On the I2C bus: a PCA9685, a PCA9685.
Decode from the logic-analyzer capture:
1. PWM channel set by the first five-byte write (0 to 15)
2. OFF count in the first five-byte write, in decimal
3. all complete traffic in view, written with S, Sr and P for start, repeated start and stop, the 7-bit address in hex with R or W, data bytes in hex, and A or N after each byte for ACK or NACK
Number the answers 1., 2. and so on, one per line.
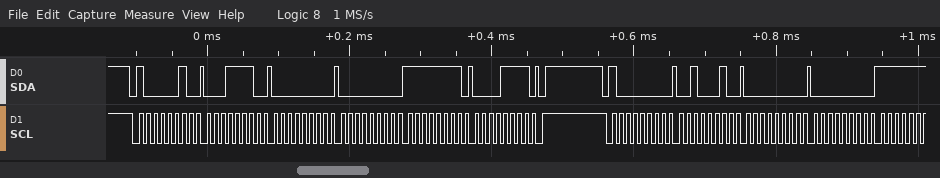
1. 6
2. 4095
3. S 41W A 1E A 00 A 00 A FF A 0F A P S 40W A 22 A 00 A 00 A
